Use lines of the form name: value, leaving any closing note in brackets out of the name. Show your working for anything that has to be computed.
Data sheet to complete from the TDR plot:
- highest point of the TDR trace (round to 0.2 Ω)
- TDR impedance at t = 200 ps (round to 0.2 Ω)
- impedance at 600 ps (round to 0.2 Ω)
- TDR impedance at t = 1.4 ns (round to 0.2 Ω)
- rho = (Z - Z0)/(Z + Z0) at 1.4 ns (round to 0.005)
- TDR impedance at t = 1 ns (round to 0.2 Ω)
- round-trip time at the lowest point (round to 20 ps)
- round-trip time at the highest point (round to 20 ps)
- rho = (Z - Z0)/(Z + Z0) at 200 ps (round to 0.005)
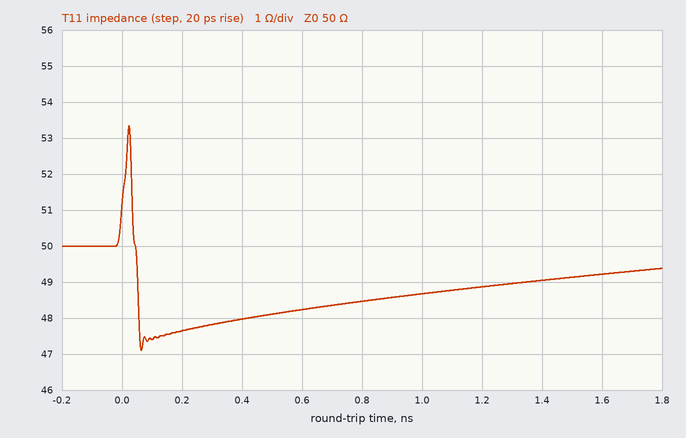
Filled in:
highest point of the TDR trace: 53.4 Ω
TDR impedance at t = 200 ps: 47.6 Ω
impedance at 600 ps: 48.2 Ω
TDR impedance at t = 1.4 ns: 49.0 Ω
rho = (Z - Z0)/(Z + Z0) at 1.4 ns: (49 − 50)/(49 + 50) ≈ -0.010
TDR impedance at t = 1 ns: 48.6 Ω
round-trip time at the lowest point: 60 ps
round-trip time at the highest point: 20 ps
rho = (Z - Z0)/(Z + Z0) at 200 ps: (47.6 − 50)/(47.6 + 50) ≈ -0.025
